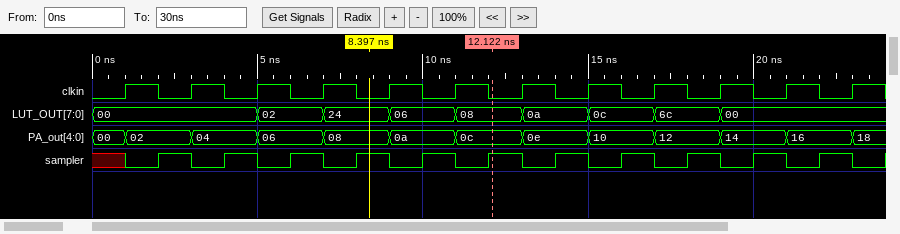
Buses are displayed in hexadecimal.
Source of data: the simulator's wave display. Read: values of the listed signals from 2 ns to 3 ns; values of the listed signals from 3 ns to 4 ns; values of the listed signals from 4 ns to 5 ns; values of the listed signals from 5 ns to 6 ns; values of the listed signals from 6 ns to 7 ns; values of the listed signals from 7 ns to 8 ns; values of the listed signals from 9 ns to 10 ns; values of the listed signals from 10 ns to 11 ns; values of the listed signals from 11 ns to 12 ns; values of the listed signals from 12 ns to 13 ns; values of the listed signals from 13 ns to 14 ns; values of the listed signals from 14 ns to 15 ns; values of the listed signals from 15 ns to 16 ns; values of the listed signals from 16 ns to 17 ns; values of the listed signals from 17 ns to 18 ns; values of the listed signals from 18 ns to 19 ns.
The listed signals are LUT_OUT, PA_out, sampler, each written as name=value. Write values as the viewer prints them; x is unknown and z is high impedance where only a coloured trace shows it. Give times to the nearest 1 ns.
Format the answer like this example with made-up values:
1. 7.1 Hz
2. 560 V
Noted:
1. LUT_OUT=00, PA_out=02, sampler=1
2. LUT_OUT=00, PA_out=04, sampler=0
3. LUT_OUT=00, PA_out=04, sampler=1
4. LUT_OUT=02, PA_out=06, sampler=0
5. LUT_OUT=02, PA_out=06, sampler=1
6. LUT_OUT=24, PA_out=08, sampler=0
7. LUT_OUT=06, PA_out=0a, sampler=0
8. LUT_OUT=06, PA_out=0a, sampler=1
9. LUT_OUT=08, PA_out=0c, sampler=0
10. LUT_OUT=08, PA_out=0c, sampler=1
11. LUT_OUT=0a, PA_out=0e, sampler=0
12. LUT_OUT=0a, PA_out=0e, sampler=1
13. LUT_OUT=0c, PA_out=10, sampler=0
14. LUT_OUT=0c, PA_out=10, sampler=1
15. LUT_OUT=6c, PA_out=12, sampler=0
16. LUT_OUT=6c, PA_out=12, sampler=1
